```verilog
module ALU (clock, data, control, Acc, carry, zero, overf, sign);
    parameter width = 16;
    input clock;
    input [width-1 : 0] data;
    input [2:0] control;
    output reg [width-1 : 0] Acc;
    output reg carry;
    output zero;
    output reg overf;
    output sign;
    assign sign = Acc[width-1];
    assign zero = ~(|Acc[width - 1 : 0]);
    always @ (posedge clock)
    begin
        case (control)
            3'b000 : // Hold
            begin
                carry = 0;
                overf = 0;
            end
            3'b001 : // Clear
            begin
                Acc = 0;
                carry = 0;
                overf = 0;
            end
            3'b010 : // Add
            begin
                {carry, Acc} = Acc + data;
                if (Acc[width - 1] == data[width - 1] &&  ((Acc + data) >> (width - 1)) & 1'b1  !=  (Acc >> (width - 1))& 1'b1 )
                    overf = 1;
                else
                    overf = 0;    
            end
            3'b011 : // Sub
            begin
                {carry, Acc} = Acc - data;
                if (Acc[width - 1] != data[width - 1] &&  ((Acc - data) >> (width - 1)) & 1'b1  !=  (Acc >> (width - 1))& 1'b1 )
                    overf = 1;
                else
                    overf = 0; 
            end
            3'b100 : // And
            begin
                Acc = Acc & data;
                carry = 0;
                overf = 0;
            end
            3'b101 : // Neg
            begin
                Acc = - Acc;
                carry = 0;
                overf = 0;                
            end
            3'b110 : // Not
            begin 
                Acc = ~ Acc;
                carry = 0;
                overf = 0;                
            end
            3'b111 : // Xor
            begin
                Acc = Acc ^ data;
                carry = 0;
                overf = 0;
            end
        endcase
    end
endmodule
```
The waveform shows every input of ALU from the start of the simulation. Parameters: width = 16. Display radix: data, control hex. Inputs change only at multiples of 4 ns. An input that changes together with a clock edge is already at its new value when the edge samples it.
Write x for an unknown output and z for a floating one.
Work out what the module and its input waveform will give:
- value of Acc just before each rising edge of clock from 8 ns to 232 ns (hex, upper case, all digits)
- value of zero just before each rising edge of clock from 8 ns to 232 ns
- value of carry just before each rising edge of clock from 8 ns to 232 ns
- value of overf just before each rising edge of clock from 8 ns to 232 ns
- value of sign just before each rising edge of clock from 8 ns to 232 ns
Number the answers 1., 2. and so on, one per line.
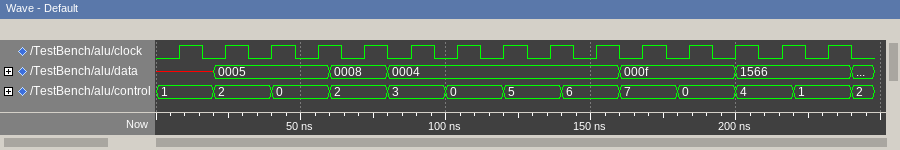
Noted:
1. x, 0000, 0005, 0005, 0005, 000D, 0009, 0009, FFF7, 0009, FFF6, FFF9, FFF9, 1560, 1560
2. x 1 0 0 0 0 0 0 0 0 0 0 0 0 0
3. x 0 0 0 0 0 0 0 0 0 0 0 0 0 0
4. x 0 0 0 0 0 0 0 0 0 0 0 0 0 0
5. x 0 0 0 0 0 0 0 1 0 1 1 1 0 0
